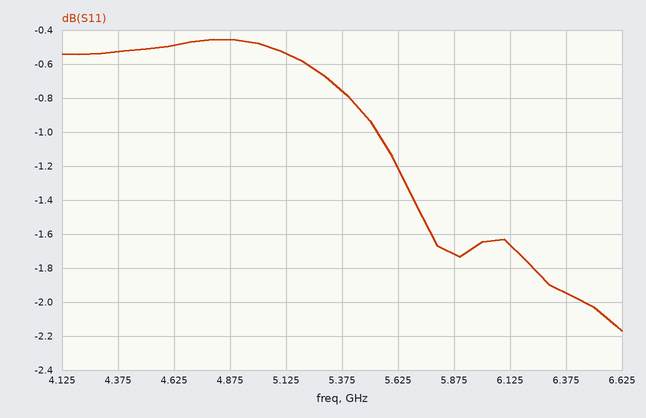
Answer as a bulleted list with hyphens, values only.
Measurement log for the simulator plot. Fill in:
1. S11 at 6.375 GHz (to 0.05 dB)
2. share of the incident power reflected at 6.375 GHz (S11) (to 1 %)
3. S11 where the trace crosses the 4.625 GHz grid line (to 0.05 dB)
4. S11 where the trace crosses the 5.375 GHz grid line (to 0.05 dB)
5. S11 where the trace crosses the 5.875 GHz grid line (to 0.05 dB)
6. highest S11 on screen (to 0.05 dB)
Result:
- -1.95 dB
- 64 %
- -0.50 dB
- -0.75 dB
- -1.70 dB
- -0.45 dB
